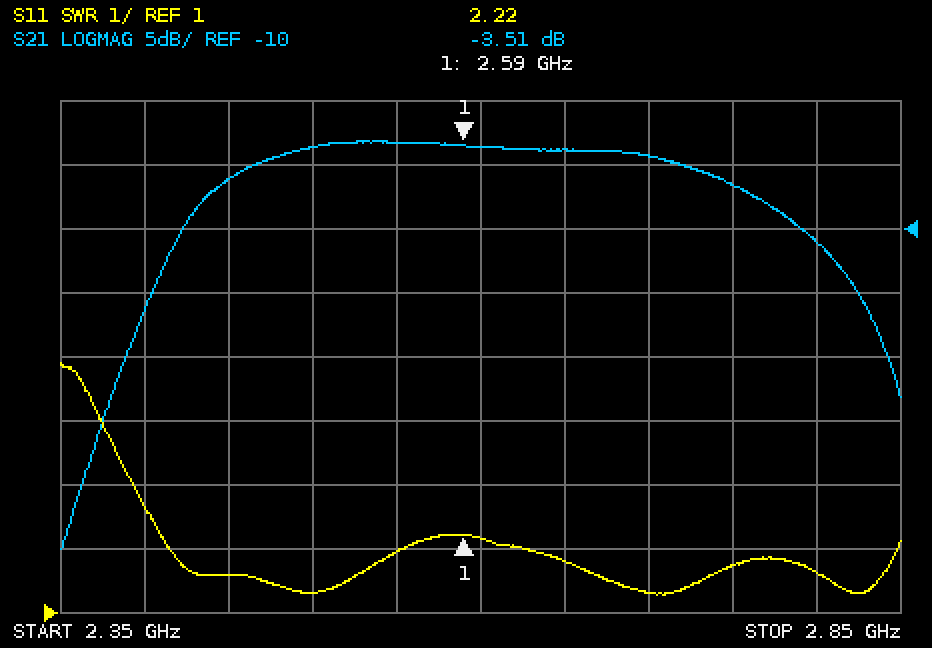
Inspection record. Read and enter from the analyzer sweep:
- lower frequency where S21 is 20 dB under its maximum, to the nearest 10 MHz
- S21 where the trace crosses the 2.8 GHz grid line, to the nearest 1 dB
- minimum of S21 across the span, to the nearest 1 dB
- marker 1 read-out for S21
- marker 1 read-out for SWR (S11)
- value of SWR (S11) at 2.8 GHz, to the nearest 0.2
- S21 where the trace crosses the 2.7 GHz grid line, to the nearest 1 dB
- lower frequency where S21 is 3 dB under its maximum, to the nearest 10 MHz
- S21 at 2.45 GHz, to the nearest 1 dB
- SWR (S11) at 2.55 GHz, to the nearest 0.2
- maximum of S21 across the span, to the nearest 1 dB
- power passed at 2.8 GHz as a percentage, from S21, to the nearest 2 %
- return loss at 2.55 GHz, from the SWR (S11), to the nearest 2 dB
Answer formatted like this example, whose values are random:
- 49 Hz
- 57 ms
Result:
- 2.38 GHz
- -11 dB
- -35 dB
- -3.51 dB
- 2.22
- 1.6
- -4 dB
- 2.45 GHz
- -6 dB
- 2.0
- -3 dB
- 8 %
- 10 dB
